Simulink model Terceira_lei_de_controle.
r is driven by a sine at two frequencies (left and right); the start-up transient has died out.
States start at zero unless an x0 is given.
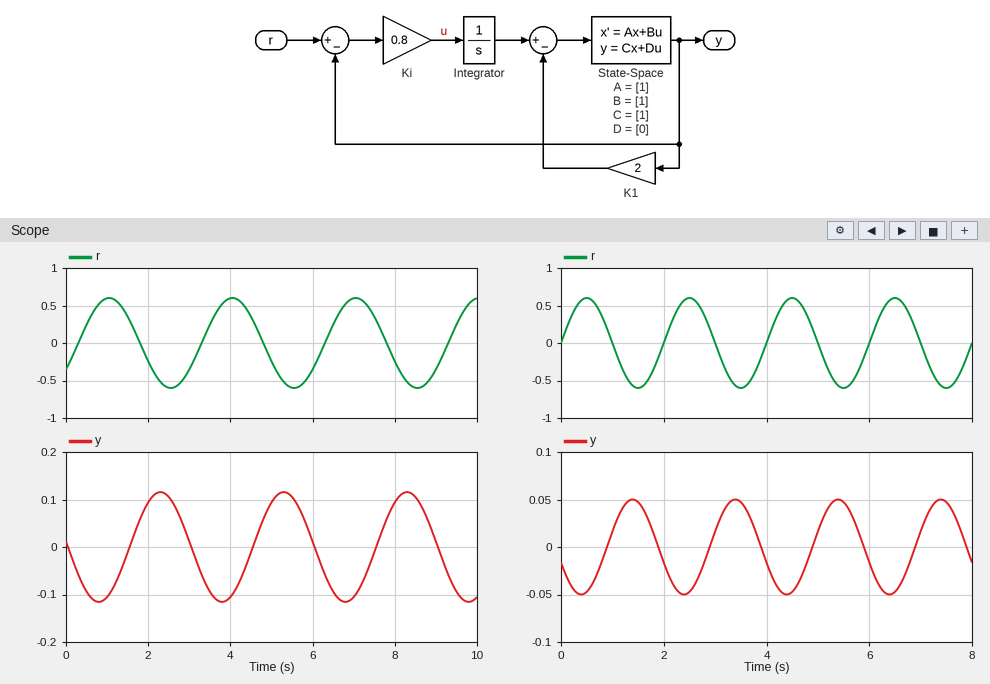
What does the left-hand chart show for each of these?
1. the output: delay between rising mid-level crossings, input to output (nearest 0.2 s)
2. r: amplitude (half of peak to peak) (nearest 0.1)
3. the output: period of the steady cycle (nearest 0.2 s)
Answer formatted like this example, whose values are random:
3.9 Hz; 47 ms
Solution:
1.2 s; 0.6; 3.0 s
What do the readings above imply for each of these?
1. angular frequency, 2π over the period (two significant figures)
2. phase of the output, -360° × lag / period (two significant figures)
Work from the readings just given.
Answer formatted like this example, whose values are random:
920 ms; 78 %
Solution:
2.1 rad/s; -140°
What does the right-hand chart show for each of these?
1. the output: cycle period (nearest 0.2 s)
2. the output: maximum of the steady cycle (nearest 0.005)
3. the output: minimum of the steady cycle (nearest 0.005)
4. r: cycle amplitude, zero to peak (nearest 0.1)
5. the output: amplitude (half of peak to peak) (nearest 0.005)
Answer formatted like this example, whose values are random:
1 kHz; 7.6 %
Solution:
2.0 s; 0.050; -0.050; 0.6; 0.050
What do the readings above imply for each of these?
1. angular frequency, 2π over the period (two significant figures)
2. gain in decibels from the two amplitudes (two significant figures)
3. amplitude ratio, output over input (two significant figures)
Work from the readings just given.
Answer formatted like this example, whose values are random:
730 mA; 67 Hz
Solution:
3.1 rad/s; -22 dB; 0.083
